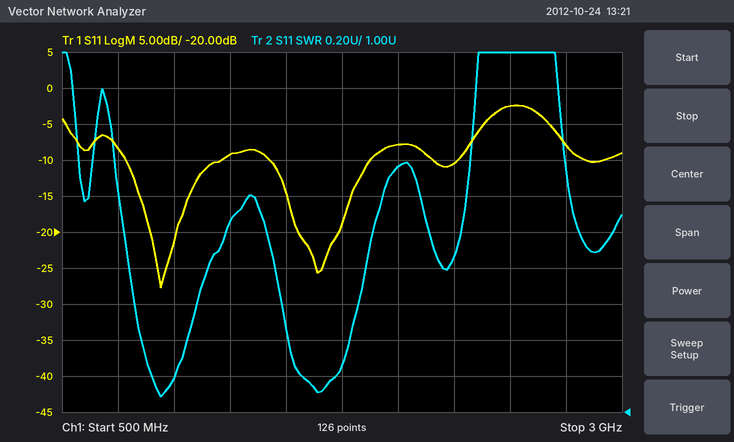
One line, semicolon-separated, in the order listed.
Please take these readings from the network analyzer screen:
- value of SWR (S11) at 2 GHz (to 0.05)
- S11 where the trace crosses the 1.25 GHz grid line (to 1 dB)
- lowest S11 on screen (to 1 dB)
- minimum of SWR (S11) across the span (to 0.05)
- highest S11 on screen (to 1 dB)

2.35; -9 dB; -28 dB; 1.10; -2 dB
